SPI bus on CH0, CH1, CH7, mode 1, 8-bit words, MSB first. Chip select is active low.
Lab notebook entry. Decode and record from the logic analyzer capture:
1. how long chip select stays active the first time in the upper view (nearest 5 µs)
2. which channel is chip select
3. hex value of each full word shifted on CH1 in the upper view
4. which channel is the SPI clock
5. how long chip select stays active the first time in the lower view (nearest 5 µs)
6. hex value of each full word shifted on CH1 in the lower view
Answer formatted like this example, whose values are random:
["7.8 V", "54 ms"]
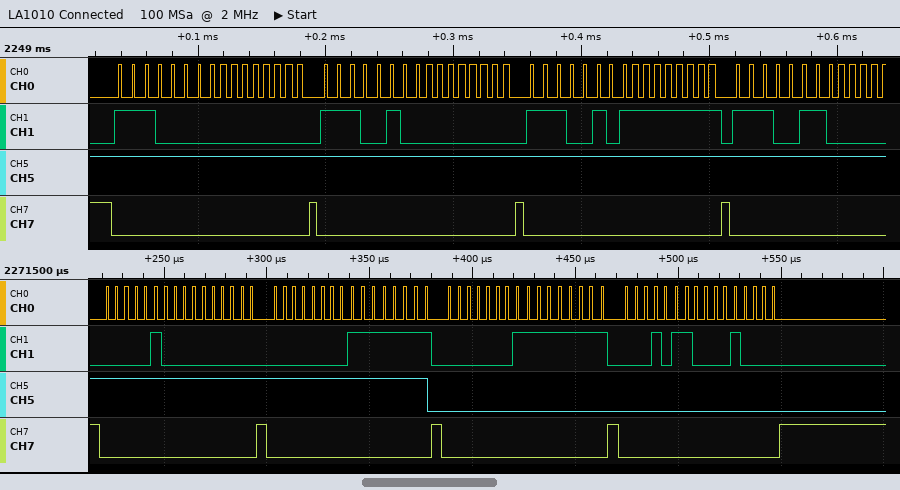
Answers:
["155 µs", "CH7", "E0, 00, E4, 00, E5, FF, E6", "CH0", "75 µs", "04, 00, 00, FF, 01, FF, 16, 10"]
